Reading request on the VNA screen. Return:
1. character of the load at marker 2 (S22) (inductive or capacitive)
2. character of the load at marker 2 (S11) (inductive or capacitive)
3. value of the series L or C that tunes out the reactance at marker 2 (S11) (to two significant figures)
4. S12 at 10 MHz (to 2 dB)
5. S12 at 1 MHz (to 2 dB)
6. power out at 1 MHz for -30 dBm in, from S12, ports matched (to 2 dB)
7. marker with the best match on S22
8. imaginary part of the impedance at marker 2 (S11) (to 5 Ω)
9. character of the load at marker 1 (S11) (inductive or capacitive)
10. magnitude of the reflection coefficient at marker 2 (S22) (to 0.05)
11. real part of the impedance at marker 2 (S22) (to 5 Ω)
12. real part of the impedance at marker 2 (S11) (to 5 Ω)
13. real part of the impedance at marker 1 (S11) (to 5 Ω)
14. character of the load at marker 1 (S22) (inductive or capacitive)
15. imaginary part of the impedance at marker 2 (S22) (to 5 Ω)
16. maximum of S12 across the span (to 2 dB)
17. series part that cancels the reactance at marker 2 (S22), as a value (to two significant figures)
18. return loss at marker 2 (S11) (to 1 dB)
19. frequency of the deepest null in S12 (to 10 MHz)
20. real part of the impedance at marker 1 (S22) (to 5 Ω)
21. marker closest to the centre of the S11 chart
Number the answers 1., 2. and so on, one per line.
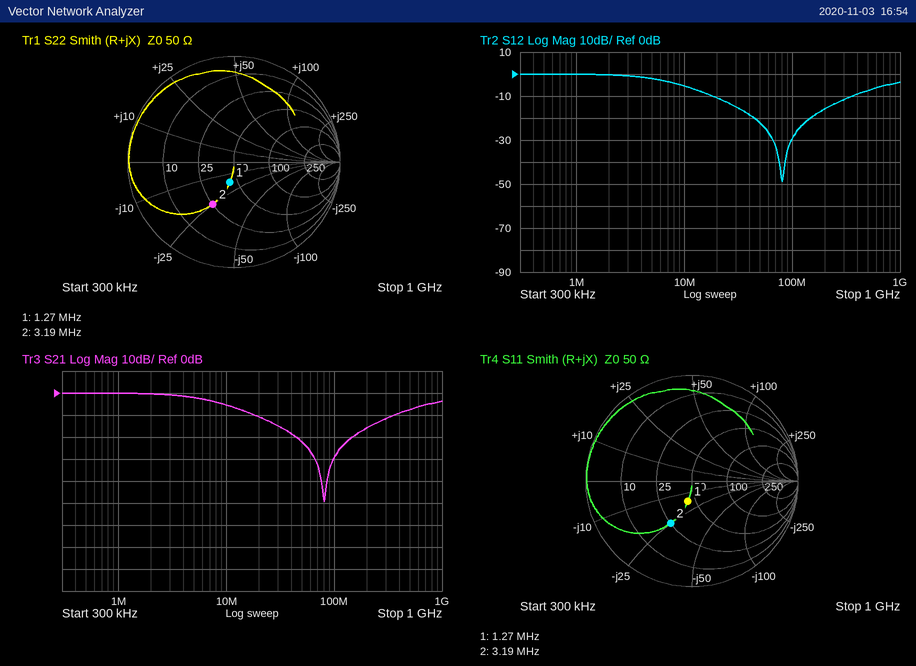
1. capacitive
2. capacitive
3. 1.2 µH
4. -6 dB
5. 0 dB
6. -30 dBm
7. marker 1
8. -25 Ω
9. capacitive
10. 0.45
11. 25 Ω
12. 25 Ω
13. 45 Ω
14. capacitive
15. -25 Ω
16. 0 dB
17. 1.2 µH
18. 7 dB
19. 80 MHz
20. 45 Ω
21. marker 1
